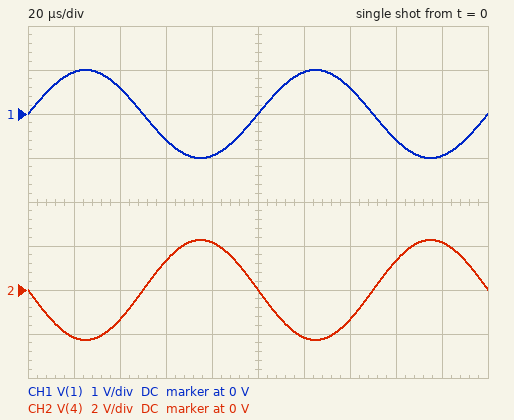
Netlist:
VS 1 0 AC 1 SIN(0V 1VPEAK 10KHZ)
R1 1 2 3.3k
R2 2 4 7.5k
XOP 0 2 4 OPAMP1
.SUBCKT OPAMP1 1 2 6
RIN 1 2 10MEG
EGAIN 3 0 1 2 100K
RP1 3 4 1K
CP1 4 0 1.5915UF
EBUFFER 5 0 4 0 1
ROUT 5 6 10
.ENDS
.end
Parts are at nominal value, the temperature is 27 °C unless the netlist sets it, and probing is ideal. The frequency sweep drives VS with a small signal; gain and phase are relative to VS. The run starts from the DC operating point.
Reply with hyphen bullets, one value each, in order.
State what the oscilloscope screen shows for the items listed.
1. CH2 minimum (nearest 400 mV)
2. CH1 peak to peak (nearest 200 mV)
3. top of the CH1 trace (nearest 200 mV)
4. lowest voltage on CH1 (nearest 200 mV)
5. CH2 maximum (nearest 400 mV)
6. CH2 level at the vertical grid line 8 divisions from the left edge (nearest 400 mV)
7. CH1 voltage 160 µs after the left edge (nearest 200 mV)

- -2.4 V
- 2.0 V
- 1.0 V
- -1.0 V
- 2.4 V
- 1.2 V
- -600 mV
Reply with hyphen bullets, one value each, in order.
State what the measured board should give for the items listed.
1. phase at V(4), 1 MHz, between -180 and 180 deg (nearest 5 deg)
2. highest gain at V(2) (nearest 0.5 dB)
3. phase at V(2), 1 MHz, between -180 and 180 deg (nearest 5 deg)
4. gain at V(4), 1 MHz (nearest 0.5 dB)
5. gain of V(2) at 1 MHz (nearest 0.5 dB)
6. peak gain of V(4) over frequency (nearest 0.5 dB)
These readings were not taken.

- 160 deg
- -3.0 dB
- 70 deg
- 6.5 dB
- -13.5 dB
- 7.0 dB
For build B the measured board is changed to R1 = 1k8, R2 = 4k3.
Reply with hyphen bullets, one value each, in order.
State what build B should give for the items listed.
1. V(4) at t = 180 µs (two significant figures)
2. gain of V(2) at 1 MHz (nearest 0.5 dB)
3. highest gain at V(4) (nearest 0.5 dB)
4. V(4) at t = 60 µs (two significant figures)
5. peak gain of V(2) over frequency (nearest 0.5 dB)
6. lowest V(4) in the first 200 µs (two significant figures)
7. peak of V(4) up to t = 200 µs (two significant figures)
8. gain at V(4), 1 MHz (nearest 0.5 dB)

- 2.3 V
- -13.0 dB
- 7.5 dB
- 1.4 V
- -3.0 dB
- -2.4 V
- 2.4 V
- 7.0 dB
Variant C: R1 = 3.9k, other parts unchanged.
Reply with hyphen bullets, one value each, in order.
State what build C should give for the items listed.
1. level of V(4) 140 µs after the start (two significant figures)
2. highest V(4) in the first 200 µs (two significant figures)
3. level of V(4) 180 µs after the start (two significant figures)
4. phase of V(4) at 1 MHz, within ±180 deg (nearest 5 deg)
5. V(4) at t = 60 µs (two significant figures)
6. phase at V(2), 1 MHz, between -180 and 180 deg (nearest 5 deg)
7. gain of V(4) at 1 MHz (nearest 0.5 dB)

- -1.1 V
- 1.9 V
- 1.8 V
- 165 deg
- 1.1 V
- 75 deg
- 5.5 dB
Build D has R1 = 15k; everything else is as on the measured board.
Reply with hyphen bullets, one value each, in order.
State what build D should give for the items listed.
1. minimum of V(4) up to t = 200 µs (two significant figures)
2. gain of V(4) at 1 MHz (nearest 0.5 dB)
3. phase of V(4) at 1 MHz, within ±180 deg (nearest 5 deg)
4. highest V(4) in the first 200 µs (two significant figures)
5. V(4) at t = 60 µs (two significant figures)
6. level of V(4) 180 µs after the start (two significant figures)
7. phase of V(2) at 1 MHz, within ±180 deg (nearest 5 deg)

- -500 mV
- -6.0 dB
- 170 deg
- 500 mV
- 290 mV
- 480 mV
- 80 deg
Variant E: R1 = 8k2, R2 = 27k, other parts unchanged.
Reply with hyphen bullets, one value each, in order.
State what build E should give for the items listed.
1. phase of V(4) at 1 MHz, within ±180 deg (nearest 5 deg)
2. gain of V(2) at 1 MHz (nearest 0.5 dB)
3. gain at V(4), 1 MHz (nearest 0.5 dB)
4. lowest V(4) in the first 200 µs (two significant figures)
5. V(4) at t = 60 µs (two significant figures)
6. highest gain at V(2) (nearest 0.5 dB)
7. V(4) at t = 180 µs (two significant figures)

- 155 deg
- -10.5 dB
- 9.5 dB
- -3.3 V
- 1.9 V
- -2.5 dB
- 3.1 V
